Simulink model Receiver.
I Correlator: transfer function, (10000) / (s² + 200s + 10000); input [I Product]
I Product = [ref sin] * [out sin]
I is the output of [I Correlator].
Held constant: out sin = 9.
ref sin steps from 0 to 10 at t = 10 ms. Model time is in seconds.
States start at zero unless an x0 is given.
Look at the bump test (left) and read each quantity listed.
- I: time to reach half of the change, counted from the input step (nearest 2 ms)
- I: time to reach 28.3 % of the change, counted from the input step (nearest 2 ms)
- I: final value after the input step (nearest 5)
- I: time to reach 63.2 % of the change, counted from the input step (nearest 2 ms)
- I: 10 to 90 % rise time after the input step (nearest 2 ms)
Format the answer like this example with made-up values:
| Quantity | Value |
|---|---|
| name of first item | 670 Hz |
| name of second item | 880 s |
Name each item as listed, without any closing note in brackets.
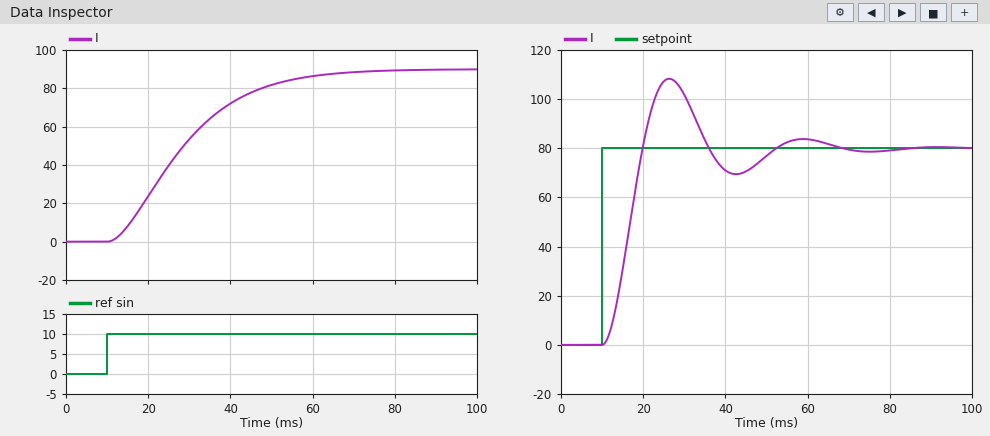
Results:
| Quantity | Value |
|---|---|
| I: time to reach half of the change, counted from the input step | 16 ms |
| I: time to reach 28.3 % of the change, counted from the input step | 10 ms |
| I: final value after the input step | 90 |
| I: time to reach 63.2 % of the change, counted from the input step | 22 ms |
| I: 10 to 90 % rise time after the input step | 34 ms |
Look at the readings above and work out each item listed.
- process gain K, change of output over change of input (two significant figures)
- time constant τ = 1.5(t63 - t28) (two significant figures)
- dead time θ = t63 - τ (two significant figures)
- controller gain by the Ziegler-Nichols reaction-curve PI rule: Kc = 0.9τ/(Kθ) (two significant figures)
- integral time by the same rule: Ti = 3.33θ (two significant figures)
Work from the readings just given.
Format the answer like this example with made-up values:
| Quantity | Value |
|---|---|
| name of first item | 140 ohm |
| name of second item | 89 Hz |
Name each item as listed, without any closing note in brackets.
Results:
| Quantity | Value |
|---|---|
| process gain K, change of output over change of input | 9.0 |
| time constant τ = 1.5(t63 - t28) | 18 ms |
| dead time θ = t63 - τ | 4.0 ms |
| controller gain by the Ziegler-Nichols reaction-curve PI rule: Kc = 0.9τ/(Kθ) | 0.45 |
| integral time by the same rule: Ti = 3.33θ | 13 ms |
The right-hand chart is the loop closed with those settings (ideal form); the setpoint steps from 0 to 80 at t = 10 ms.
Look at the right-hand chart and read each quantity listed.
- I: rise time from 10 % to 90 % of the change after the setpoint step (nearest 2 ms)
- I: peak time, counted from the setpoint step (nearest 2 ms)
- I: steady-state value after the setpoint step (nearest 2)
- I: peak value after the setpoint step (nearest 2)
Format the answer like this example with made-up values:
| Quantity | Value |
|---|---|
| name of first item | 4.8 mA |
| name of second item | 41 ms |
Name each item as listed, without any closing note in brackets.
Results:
| Quantity | Value |
|---|---|
| I: rise time from 10 % to 90 % of the change after the setpoint step | 6 ms |
| I: peak time, counted from the setpoint step | 16 ms |
| I: steady-state value after the setpoint step | 80 |
| I: peak value after the setpoint step | 108 |
